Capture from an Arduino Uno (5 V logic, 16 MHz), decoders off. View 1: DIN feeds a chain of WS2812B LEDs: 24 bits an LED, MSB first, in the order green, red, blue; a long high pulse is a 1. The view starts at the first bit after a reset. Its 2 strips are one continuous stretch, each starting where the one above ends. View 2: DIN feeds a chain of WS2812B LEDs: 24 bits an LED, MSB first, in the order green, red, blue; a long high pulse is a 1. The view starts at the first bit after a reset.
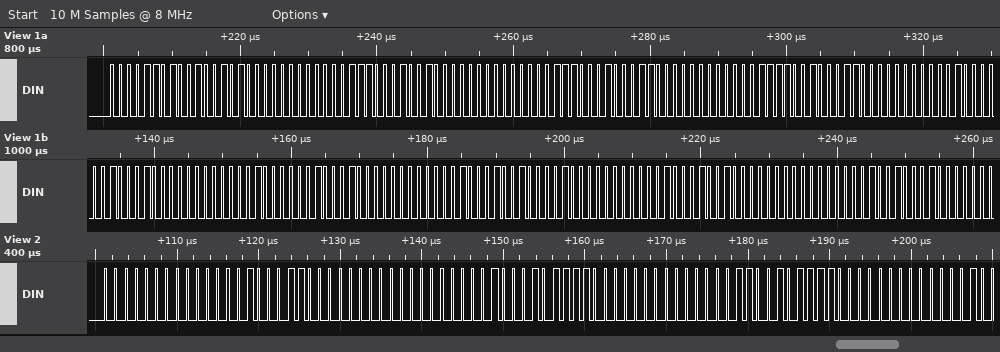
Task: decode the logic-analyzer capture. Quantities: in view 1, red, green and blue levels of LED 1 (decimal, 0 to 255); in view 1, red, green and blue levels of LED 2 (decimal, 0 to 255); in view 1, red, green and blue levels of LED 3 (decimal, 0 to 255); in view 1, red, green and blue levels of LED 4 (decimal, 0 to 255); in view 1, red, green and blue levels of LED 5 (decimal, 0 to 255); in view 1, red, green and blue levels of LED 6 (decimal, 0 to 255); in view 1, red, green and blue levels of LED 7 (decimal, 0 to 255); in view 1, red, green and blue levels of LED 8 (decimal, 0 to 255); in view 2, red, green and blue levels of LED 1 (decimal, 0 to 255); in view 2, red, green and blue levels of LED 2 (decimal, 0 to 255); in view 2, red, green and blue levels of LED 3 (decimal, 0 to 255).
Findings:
37, 13, 0
36, 14, 0
35, 14, 0
35, 15, 0
34, 16, 0
34, 16, 0
33, 17, 0
32, 17, 0
2, 0, 48
2, 0, 47
3, 0, 47
